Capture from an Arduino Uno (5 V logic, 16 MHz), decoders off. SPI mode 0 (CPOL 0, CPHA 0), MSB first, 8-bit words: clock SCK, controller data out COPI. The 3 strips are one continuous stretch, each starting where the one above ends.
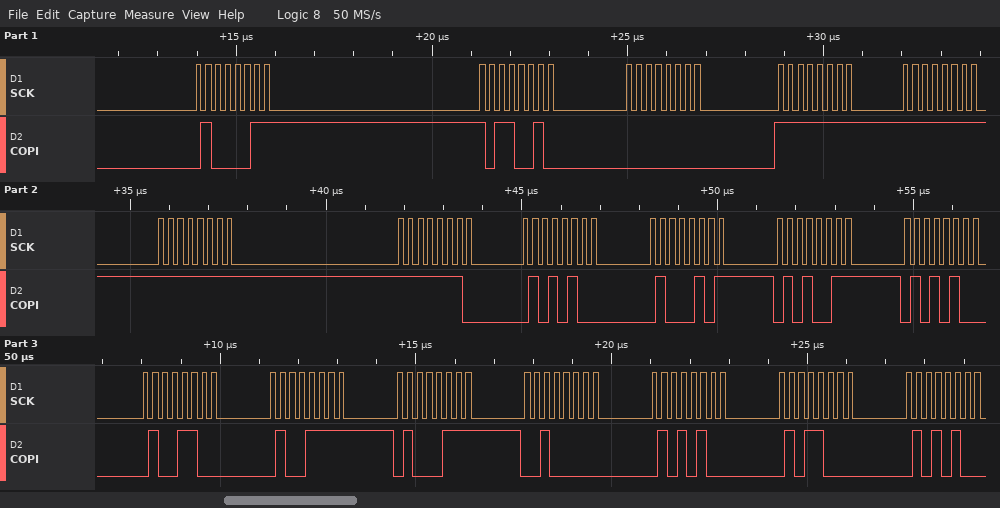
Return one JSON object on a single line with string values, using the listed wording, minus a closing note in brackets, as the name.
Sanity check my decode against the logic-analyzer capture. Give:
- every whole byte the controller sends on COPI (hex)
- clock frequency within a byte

{"every whole byte the controller sends on COPI": "43 B2 00 FF FF FF FE 54 45 53 54 4C 4F 47 20 54 58 54", "clock frequency within a byte": "4 MHz"}
